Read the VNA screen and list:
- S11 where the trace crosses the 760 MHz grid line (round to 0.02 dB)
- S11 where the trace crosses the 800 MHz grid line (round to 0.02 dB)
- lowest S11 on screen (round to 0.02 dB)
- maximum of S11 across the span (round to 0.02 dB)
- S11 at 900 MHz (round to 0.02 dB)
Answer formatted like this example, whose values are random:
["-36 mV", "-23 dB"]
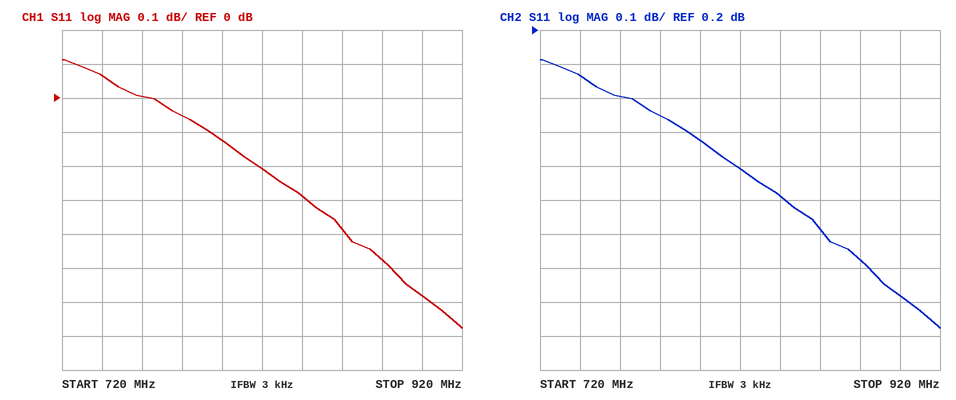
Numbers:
["0.00 dB", "-0.12 dB", "-0.68 dB", "0.12 dB", "-0.58 dB"]
